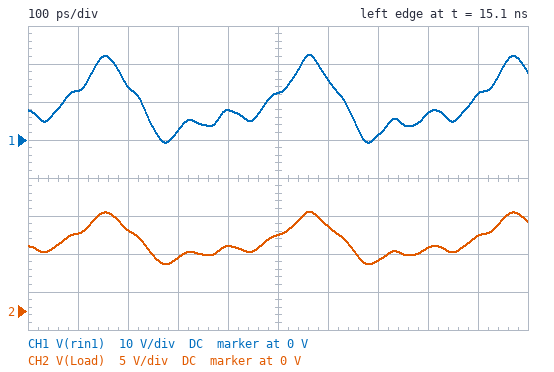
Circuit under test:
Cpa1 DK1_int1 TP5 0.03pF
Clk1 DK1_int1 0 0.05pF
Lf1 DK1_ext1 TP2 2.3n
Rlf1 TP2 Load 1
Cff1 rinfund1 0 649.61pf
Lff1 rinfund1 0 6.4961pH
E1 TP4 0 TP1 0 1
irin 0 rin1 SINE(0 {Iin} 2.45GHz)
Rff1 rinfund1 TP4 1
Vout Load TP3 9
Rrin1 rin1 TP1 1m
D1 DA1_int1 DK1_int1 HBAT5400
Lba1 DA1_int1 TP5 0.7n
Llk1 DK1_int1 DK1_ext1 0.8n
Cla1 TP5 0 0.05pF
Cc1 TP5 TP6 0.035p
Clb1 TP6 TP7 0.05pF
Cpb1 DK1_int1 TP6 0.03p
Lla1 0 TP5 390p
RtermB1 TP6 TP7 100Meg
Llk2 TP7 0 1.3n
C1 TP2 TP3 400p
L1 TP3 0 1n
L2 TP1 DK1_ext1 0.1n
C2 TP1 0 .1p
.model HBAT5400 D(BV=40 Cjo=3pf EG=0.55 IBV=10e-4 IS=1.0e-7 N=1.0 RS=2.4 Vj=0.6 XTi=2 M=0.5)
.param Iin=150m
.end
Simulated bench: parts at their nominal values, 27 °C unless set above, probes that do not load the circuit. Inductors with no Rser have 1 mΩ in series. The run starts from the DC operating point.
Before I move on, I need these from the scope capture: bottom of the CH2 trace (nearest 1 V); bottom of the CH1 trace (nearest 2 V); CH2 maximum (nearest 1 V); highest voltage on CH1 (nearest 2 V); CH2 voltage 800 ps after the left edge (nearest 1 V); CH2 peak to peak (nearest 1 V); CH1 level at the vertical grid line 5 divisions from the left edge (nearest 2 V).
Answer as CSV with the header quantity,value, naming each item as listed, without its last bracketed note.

quantity,value
bottom of the CH2 trace,6 V
bottom of the CH1 trace,0 V
CH2 maximum,13 V
highest voltage on CH1,22 V
CH2 voltage 800 ps after the left edge,8 V
CH2 peak to peak,7 V
CH1 level at the vertical grid line 5 divisions from the left edge,12 V
